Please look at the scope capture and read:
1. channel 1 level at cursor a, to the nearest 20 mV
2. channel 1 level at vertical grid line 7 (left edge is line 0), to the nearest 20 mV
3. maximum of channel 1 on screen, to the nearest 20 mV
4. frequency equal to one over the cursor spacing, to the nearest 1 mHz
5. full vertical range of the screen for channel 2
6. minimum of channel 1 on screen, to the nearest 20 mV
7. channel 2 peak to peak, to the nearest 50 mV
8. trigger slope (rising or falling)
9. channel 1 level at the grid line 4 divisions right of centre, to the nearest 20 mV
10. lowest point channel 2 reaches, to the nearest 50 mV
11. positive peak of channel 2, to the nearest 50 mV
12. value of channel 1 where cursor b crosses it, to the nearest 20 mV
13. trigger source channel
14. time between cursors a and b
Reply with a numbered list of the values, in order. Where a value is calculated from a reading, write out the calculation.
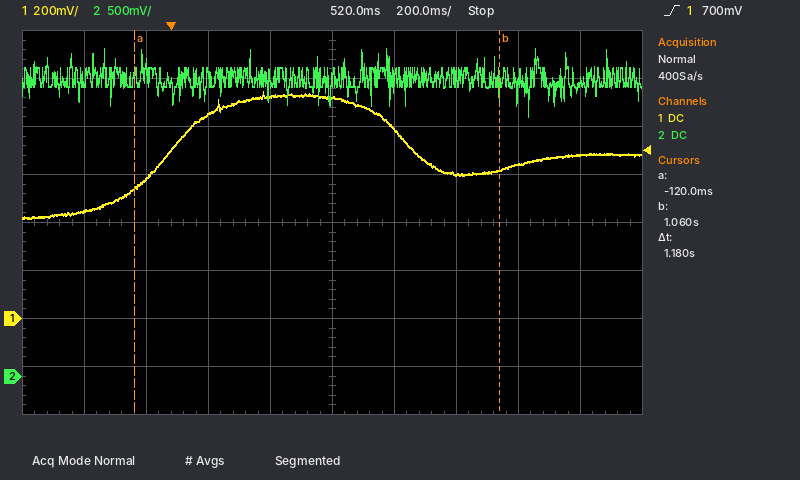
1. 540 mV
2. 600 mV
3. 940 mV
4. 1 / 1.18 s ≈ 847 mHz
5. 4 V
6. 420 mV
7. 3.40 V − (2.70 V) = 700 mV
8. rising
9. 680 mV
10. 2.70 V
11. 3.40 V
12. 620 mV
13. channel 1
14. 1.18 s
